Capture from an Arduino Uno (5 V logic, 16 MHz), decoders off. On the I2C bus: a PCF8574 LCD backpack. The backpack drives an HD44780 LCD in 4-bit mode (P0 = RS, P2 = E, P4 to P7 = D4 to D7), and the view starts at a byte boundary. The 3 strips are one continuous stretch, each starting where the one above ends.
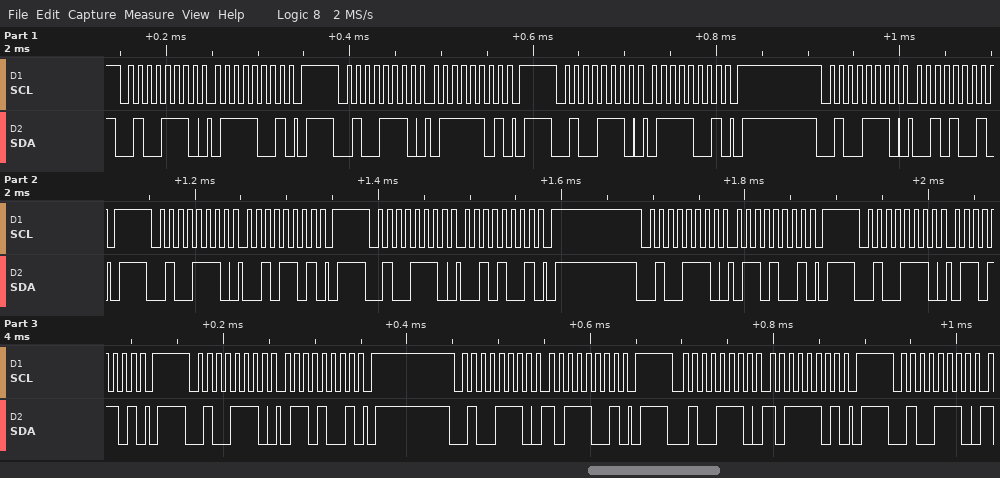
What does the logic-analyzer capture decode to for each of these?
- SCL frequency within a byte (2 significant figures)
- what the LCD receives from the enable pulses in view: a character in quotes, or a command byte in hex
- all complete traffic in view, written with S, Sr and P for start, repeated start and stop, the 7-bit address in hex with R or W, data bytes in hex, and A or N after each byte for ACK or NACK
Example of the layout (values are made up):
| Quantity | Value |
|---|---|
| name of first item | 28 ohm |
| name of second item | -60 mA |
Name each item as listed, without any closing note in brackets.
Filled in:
| Quantity | Value |
|---|---|
| SCL frequency within a byte | 100 kHz |
| what the LCD receives from the enable pulses in view: a character in quotes, or a command byte in hex | 'r' |
| all complete traffic in view, written with S, Sr and P for start, repeated start and stop, the 7-bit address in hex with R or W, data bytes in hex, and A or N after each byte for ACK or NACK | S 27W A 79 A P S 27W A 7D A P S 27W A 79 A P S 27W A 29 A P S 27W A 2D A P S 27W A 29 A P S 27W A 69 A P S 27W A 6D A P S 27W A 69 A P S 27W A B9 A P S 27W A BD A P S 27W A |
